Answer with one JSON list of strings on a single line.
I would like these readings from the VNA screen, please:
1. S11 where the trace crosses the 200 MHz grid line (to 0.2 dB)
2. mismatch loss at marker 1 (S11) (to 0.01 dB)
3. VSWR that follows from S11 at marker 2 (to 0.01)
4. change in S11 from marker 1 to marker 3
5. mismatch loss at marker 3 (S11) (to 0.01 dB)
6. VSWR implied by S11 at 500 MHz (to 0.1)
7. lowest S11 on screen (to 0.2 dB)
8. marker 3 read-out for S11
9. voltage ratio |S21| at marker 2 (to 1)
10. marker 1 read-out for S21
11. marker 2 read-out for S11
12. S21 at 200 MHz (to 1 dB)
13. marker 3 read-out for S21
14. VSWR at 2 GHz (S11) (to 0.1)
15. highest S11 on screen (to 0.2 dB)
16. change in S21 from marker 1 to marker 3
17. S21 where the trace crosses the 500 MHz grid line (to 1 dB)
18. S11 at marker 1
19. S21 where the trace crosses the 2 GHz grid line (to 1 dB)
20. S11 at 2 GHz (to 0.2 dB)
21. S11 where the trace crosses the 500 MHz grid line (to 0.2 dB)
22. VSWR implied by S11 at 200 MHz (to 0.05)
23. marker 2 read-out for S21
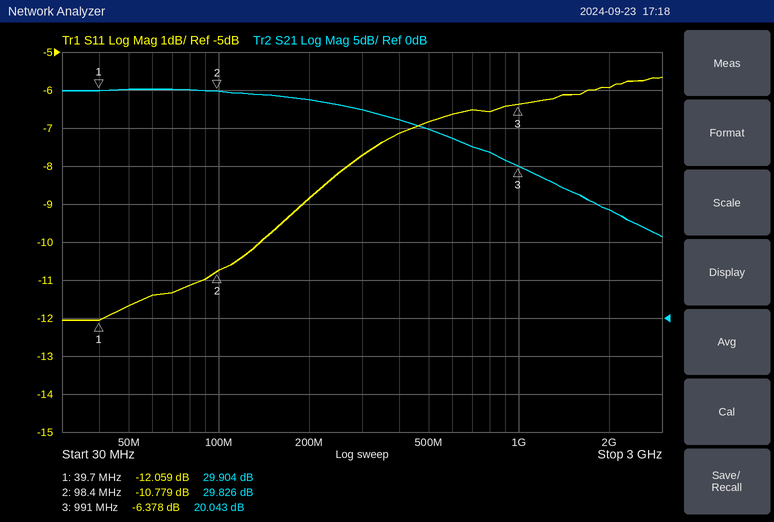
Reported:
["-8.8 dB", "0.28 dB", "1.81", "5.681 dB", "1.14 dB", "2.7", "-12.0 dB", "-6.378 dB", "31", "29.904 dB", "-10.779 dB", "29 dB", "20.043 dB", "3.0", "-5.6 dB", "-9.861 dB", "25 dB", "-12.059 dB", "14 dB", "-6.0 dB", "-6.8 dB", "2.15", "29.826 dB"]
